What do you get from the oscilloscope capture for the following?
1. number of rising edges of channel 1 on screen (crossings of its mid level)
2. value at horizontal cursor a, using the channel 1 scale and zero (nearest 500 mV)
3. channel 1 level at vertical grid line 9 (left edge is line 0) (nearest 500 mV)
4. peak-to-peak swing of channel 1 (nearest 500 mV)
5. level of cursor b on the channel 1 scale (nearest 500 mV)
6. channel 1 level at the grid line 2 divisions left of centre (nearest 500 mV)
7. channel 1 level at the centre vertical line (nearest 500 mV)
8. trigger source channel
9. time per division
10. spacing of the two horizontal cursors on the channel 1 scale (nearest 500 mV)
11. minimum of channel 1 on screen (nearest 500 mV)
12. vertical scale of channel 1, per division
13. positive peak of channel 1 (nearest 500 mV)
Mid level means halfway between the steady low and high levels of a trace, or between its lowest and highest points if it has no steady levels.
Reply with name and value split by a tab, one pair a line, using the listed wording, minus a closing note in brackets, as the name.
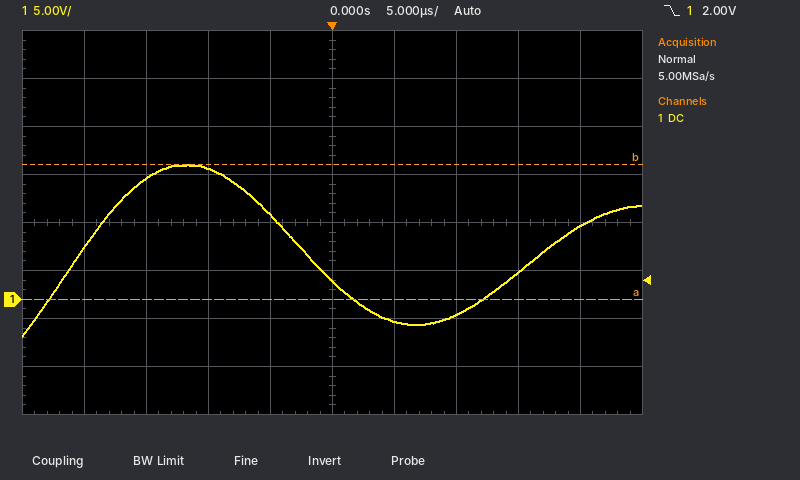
number of rising edges of channel 1 on screen	2
value at horizontal cursor a, using the channel 1 scale and zero	0.0 V
channel 1 level at vertical grid line 9 (left edge is line 0)	7.5 V
peak-to-peak swing of channel 1	18.0 V
level of cursor b on the channel 1 scale	14.0 V
channel 1 level at the grid line 2 divisions left of centre	13.5 V
channel 1 level at the centre vertical line	2.0 V
trigger source channel	channel 1
time per division	5 µs
spacing of the two horizontal cursors on the channel 1 scale	14.0 V
minimum of channel 1 on screen	-4.0 V
vertical scale of channel 1, per division	5 V
positive peak of channel 1	14.0 V
